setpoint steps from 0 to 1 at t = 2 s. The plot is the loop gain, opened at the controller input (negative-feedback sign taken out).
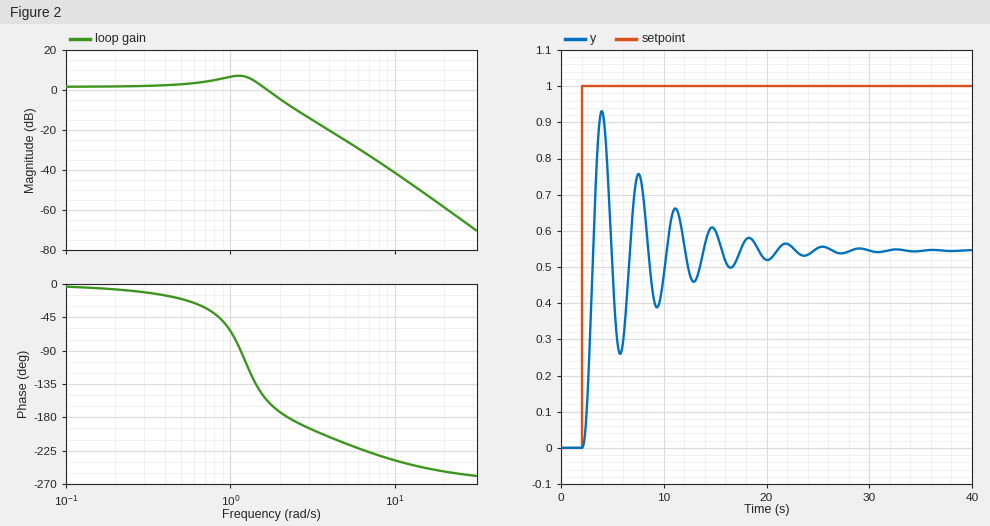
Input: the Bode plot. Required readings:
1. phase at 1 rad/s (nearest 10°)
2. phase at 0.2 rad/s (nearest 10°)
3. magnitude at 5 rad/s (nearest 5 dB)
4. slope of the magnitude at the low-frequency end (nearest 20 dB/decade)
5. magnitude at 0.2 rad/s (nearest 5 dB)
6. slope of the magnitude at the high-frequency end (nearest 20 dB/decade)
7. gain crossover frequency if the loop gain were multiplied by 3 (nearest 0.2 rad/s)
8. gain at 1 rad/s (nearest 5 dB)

-60°
-10°
-25 dB
0 dB/decade
0 dB
-60 dB/decade
2.4 rad/s
5 dB
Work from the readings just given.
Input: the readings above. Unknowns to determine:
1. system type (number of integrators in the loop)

0
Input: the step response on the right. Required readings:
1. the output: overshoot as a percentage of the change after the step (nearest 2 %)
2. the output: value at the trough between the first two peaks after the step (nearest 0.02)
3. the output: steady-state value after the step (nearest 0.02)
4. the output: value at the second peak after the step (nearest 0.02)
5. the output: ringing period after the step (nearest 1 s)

70 %
0.26
0.54
0.76
4 s
